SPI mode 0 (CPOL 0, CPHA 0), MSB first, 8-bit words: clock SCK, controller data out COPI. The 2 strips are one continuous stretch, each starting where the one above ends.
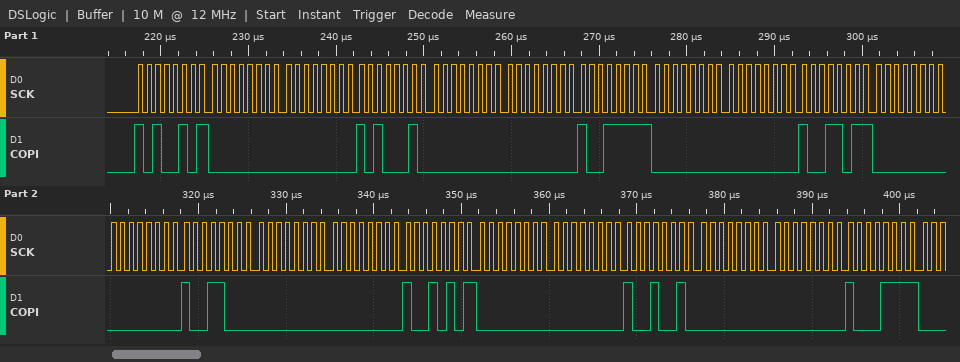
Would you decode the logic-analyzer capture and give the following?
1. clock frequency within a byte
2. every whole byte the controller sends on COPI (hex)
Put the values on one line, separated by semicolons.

1 MHz; A5 00 00 A2 00 00 9F 00 00 9B 00 00 98 00 00 95 00 00 92 00 00 8F
